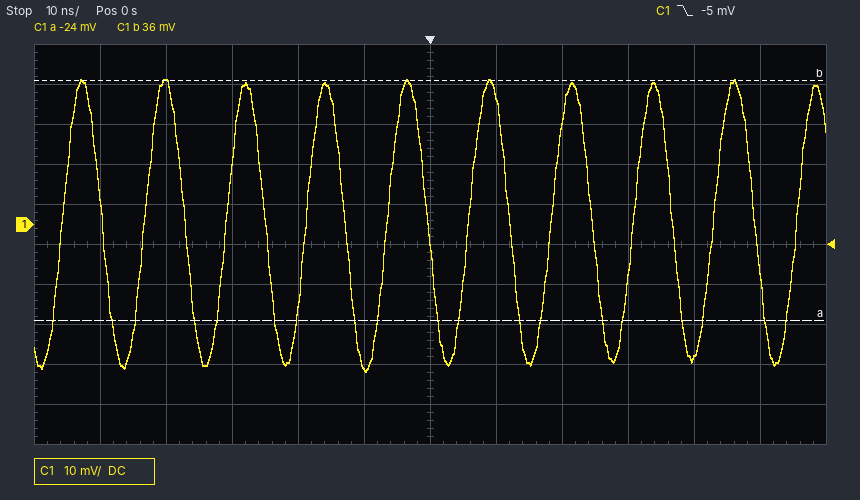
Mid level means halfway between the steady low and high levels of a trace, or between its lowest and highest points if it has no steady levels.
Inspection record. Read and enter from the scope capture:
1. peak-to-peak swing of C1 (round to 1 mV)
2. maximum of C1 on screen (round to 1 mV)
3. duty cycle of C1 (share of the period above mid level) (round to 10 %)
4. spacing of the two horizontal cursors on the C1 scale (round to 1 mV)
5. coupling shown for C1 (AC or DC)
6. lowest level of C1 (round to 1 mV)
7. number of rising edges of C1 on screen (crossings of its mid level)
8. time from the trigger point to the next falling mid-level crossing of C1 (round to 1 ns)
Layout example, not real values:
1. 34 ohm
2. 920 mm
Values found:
1. 73 mV
2. 36 mV
3. 50 %
4. 60 mV
5. DC
6. -37 mV
7. 10
8. 12 ns
